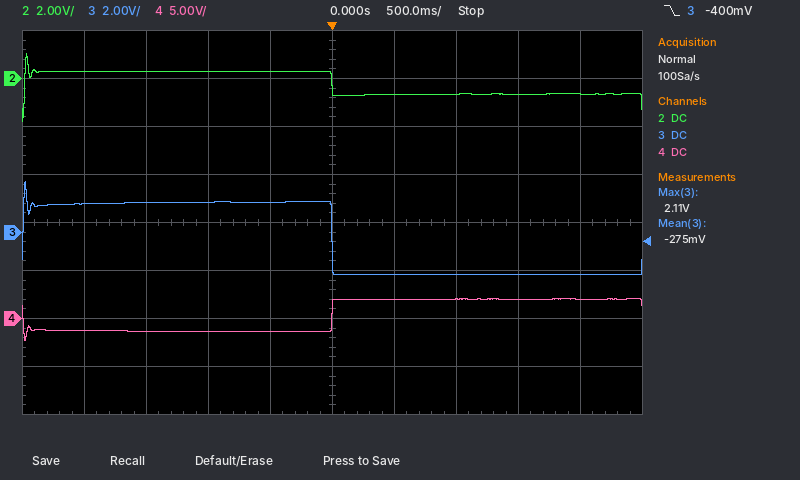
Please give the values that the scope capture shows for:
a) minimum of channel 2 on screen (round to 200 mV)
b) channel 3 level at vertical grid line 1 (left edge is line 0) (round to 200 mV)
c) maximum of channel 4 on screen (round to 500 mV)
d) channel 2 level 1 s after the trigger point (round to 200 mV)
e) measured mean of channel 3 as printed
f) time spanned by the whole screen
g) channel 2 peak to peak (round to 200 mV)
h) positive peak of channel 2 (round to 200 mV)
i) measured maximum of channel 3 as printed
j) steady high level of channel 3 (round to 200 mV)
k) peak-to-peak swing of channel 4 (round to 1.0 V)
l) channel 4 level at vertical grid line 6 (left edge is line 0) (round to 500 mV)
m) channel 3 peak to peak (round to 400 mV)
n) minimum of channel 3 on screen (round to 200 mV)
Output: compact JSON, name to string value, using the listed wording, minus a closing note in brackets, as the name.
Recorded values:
{"minimum of channel 2 on screen": "-1.8 V", "channel 3 level at vertical grid line 1 (left edge is line 0)": "1.2 V", "maximum of channel 4 on screen": "2.0 V", "channel 2 level 1 s after the trigger point": "-600 mV", "measured mean of channel 3 as printed": "-275 mV", "time spanned by the whole screen": "5 s", "channel 2 peak to peak": "2.8 V", "positive peak of channel 2": "1.0 V", "measured maximum of channel 3 as printed": "2.11 V", "steady high level of channel 3": "1.2 V", "peak-to-peak swing of channel 4": "4.0 V", "channel 4 level at vertical grid line 6 (left edge is line 0)": "2.0 V", "channel 3 peak to peak": "4.0 V", "minimum of channel 3 on screen": "-1.8 V"}
